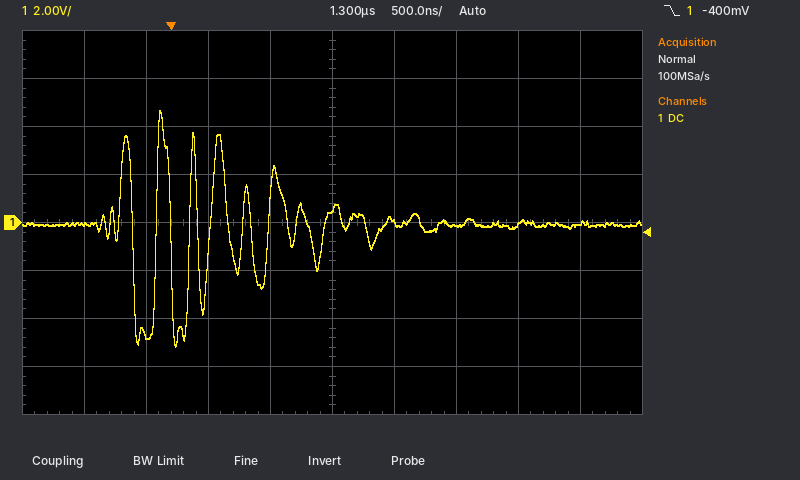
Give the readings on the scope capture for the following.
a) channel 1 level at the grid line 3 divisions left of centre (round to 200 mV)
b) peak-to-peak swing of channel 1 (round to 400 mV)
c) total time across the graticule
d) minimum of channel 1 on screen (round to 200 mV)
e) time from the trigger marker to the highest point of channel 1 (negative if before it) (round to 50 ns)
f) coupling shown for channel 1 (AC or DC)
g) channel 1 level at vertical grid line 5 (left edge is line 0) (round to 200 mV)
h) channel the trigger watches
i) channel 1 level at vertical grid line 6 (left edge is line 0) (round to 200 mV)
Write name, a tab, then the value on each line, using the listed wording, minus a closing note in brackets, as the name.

channel 1 level at the grid line 3 divisions left of centre	-4.6 V
peak-to-peak swing of channel 1	10.0 V
total time across the graticule	5 µs
minimum of channel 1 on screen	-5.2 V
time from the trigger marker to the highest point of channel 1 (negative if before it)	-100 ns
coupling shown for channel 1	DC
channel 1 level at vertical grid line 5 (left edge is line 0)	600 mV
channel the trigger watches	channel 1
channel 1 level at vertical grid line 6 (left edge is line 0)	0.0 V
